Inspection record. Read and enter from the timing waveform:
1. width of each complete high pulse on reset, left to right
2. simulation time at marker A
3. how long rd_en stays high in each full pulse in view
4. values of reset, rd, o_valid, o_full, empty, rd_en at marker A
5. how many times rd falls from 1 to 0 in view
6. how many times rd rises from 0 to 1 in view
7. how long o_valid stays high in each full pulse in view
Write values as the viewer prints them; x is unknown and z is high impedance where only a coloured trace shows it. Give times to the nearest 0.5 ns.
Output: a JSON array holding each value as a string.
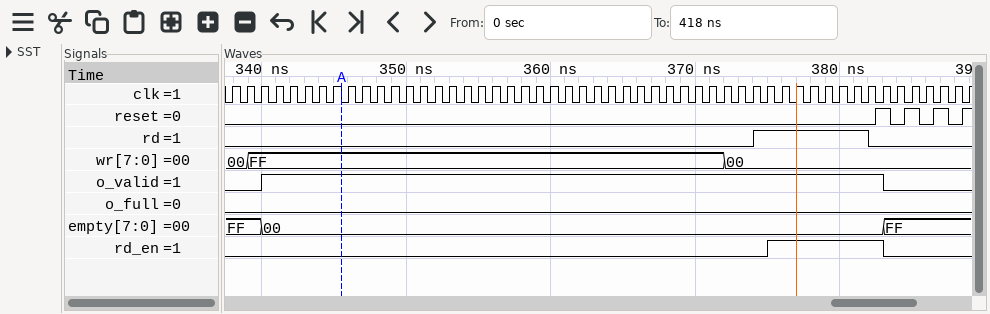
["1 ns, 1 ns, 1 ns", "345.5 ns", "8 ns", "reset=0, rd=0, o_valid=1, o_full=0, empty=00, rd_en=0", "1", "1", "43 ns"]
